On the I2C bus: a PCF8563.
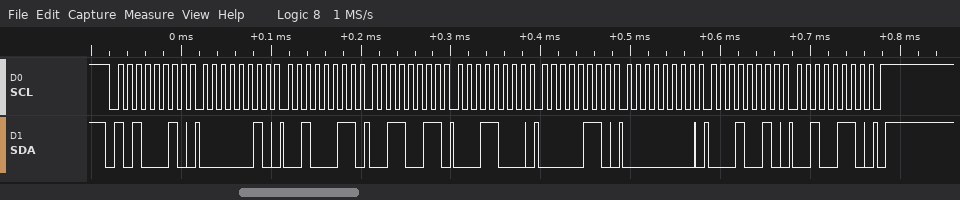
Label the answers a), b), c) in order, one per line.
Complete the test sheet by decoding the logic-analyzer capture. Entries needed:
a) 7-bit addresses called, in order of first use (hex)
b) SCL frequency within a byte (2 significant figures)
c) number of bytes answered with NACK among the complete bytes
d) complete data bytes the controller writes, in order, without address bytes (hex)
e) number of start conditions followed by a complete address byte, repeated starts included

a) 0x51
b) 100 kHz
c) 0
d) 02 23 33 18 06 00 12 26
e) 1
